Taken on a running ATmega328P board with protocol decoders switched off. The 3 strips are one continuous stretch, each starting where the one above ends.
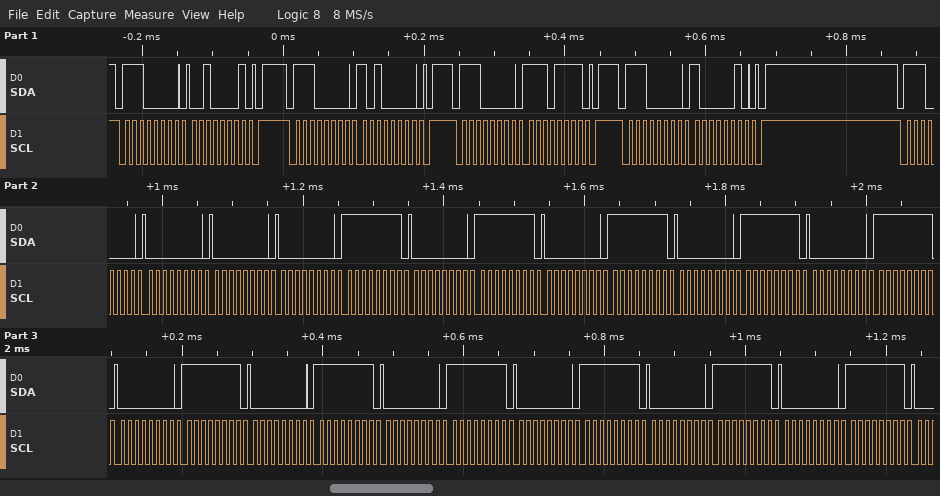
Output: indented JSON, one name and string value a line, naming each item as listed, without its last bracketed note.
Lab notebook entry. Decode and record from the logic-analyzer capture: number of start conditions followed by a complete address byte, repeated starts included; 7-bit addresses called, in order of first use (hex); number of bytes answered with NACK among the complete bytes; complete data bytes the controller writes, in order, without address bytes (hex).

{
  "number of start conditions followed by a complete address byte, repeated starts included": "5",
  "7-bit addresses called, in order of first use": "0x70",
  "number of bytes answered with NACK among the complete bytes": "0",
  "complete data bytes the controller writes, in order, without address bytes": "21 A0 EF 82 00 00 00 FF 00 FF 00 FF 00 FF 00 FF 00 FF 00 FF 00 FF 00 FF 00 FF 00 FF"
}
